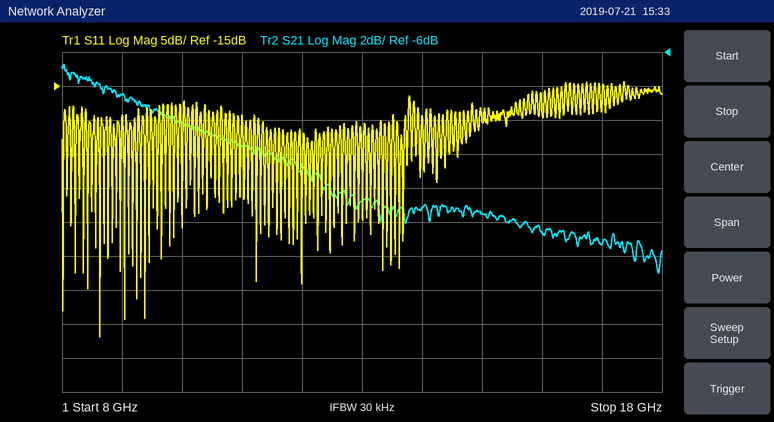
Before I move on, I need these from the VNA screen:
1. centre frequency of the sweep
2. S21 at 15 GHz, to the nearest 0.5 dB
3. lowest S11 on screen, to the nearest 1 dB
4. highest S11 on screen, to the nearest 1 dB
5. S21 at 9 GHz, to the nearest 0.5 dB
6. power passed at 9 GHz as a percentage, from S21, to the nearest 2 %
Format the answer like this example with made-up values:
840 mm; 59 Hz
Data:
13 GHz; -15.5 dB; -52 dB; -14 dB; -8.5 dB; 14 %
